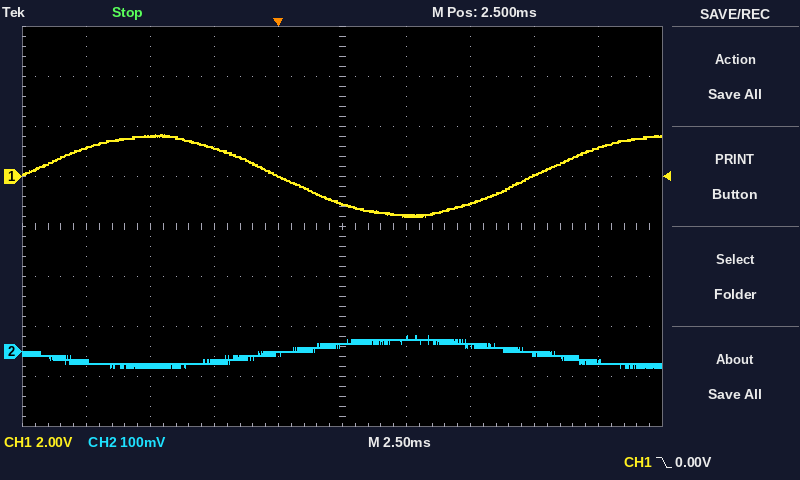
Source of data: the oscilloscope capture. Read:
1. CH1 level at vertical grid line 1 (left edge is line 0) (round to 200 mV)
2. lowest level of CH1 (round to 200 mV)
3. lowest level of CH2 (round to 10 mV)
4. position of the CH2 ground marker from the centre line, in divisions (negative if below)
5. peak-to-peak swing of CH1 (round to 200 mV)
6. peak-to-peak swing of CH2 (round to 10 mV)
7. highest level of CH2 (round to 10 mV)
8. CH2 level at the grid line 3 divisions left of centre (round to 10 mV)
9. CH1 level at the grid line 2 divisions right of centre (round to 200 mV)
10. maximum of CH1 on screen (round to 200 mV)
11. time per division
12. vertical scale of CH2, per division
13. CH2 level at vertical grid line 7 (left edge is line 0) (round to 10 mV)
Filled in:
1.2 V
-1.6 V
-30 mV
-2.5 div
3.2 V
60 mV
30 mV
-30 mV
-1.0 V
1.6 V
2.5 ms
100 mV
10 mV
